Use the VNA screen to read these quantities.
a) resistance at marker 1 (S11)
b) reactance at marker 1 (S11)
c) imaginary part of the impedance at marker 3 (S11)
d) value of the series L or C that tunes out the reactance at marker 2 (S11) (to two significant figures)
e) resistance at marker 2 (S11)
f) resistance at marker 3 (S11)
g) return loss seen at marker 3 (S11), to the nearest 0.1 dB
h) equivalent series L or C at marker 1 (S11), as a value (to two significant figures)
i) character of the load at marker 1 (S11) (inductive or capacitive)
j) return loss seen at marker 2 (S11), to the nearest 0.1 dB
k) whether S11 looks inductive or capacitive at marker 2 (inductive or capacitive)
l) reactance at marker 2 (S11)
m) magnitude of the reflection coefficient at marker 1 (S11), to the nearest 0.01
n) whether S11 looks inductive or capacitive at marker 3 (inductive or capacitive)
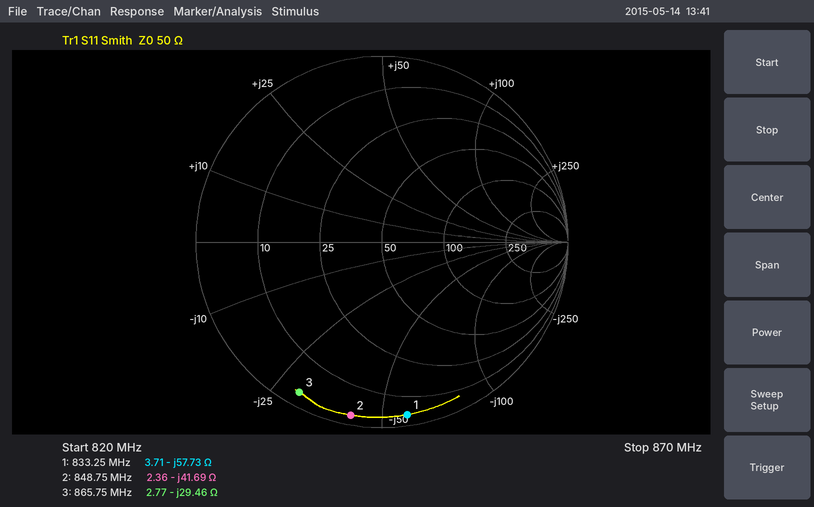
3.71 Ω
-57.73 Ω
-29.46 Ω
7.8 nH
2.36 Ω
2.77 Ω
0.7 dB
3.3 pF
capacitive
0.5 dB
capacitive
-41.69 Ω
0.94
capacitive
